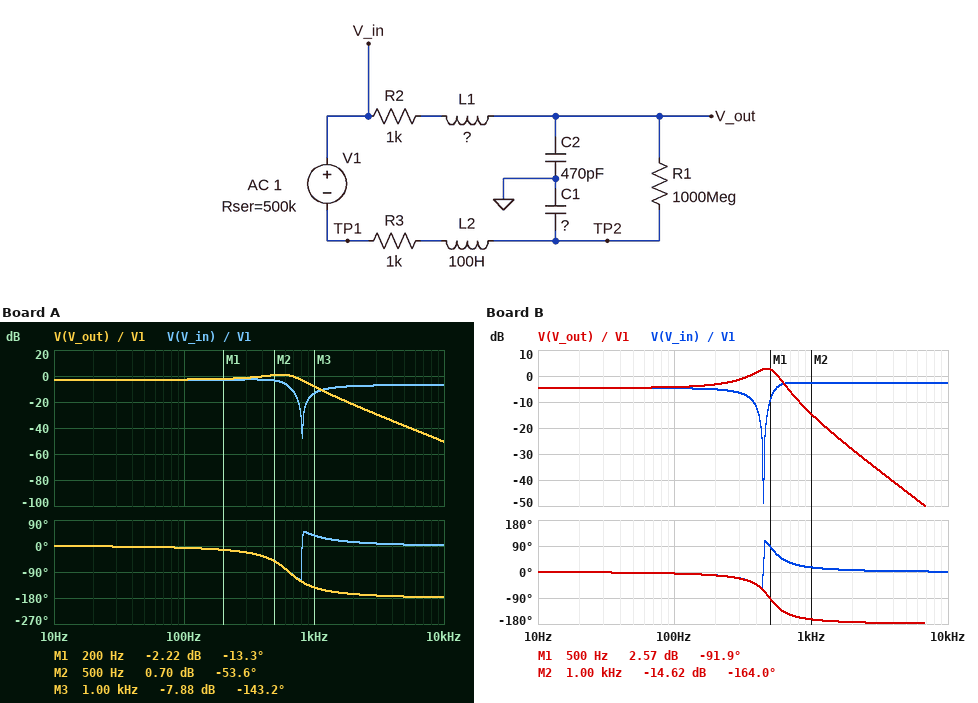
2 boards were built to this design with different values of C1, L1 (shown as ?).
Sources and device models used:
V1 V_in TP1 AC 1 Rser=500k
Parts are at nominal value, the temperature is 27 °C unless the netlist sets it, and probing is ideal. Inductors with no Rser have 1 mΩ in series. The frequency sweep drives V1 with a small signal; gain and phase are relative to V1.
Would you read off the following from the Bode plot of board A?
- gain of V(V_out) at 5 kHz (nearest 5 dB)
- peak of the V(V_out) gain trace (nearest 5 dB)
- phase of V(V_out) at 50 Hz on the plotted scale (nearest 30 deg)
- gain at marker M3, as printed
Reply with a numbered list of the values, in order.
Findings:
1. -40 dB
2. 0 dB
3. 0 deg
4. -7.88 dB
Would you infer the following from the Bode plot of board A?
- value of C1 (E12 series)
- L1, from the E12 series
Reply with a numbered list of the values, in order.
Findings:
1. 1.2 nF
2. 82 H
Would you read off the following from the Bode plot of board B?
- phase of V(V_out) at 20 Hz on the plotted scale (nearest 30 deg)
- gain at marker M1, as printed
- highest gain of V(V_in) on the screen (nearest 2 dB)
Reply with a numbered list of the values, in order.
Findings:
1. 0 deg
2. 2.57 dB
3. -2 dB
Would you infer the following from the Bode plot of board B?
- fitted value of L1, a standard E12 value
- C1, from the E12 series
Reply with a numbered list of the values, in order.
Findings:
1. 270 H
2. 680 pF
